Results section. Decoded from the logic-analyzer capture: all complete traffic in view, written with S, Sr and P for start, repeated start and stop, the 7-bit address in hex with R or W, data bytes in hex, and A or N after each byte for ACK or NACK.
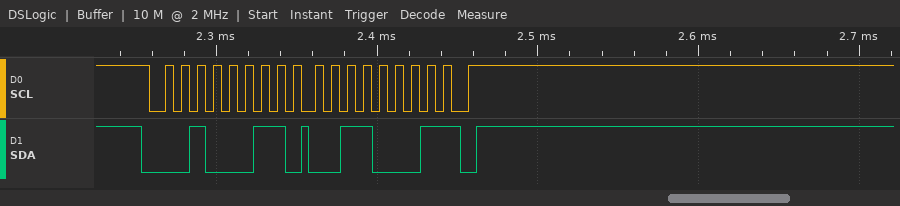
S 11R A 31 N P
